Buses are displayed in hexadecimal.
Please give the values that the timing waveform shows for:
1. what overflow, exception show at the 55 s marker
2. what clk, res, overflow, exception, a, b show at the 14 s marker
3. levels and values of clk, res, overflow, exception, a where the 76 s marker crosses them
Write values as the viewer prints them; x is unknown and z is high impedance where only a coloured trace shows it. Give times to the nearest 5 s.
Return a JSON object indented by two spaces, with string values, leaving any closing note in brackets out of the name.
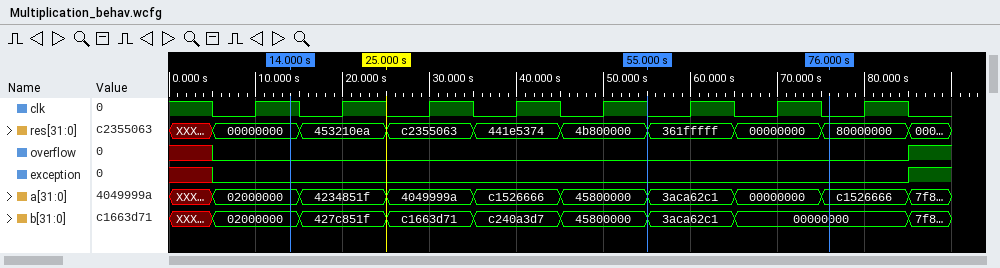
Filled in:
{
  "what overflow, exception show at the 55 s marker": "overflow=0, exception=0",
  "what clk, res, overflow, exception, a, b show at the 14 s marker": "clk=1, res=00000000, overflow=0, exception=0, a=02000000, b=02000000",
  "levels and values of clk, res, overflow, exception, a where the 76 s marker crosses them": "clk=0, res=80000000, overflow=0, exception=0, a=c1526666"
}
